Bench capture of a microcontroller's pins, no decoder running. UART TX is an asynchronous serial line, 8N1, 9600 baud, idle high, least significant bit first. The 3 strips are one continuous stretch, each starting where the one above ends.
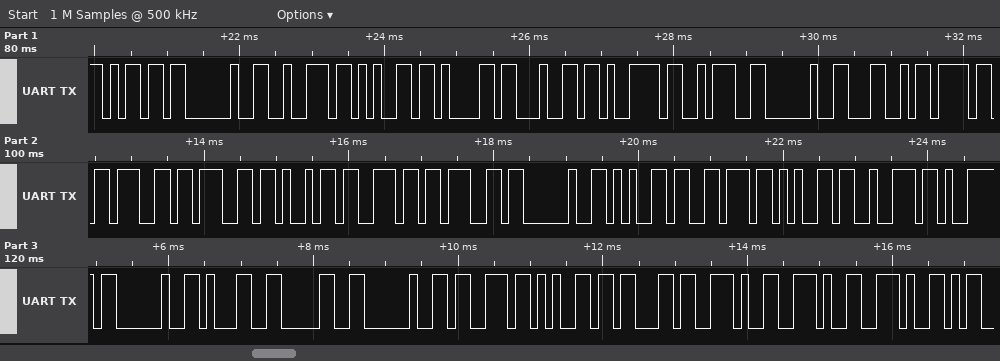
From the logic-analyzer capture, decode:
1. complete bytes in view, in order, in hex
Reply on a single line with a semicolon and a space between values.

6D 20 72 65 61 64 79 3A 20 4C 6F 67 67 69 6E 67 20 65 76 65 72 79 20 31 30 20 73 65 63 2E 2E 2E
